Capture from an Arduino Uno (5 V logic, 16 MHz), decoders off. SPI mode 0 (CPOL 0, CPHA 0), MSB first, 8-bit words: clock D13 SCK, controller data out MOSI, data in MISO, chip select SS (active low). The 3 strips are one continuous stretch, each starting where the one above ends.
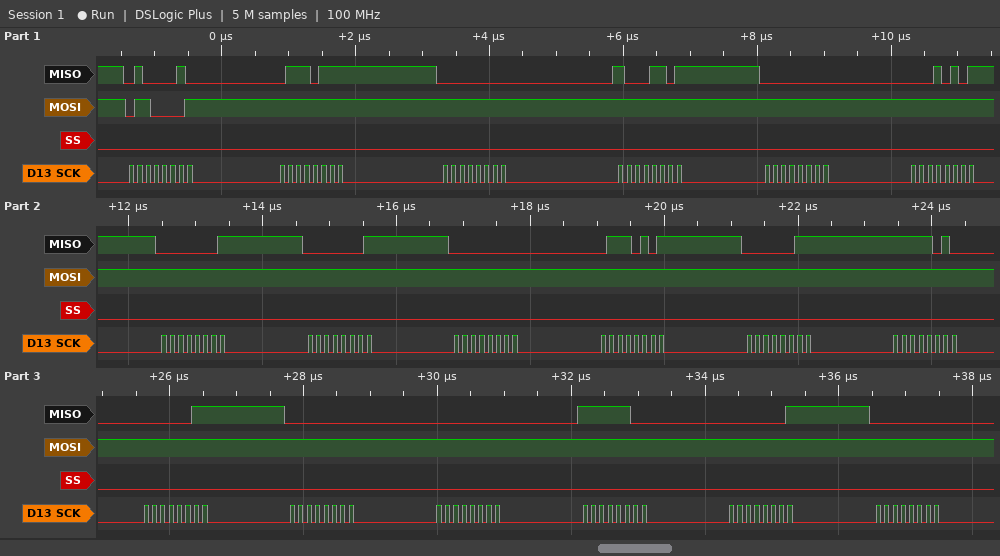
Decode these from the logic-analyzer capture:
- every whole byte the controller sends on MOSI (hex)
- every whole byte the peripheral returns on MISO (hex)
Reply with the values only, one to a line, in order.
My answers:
61 FF FF FF FF FF FF FF FF FF FF FF FF FF FF FF FF FF
42 77 00 8D 00 15 01 01 00 75 03 FA 03 00 00 FC 01 00
